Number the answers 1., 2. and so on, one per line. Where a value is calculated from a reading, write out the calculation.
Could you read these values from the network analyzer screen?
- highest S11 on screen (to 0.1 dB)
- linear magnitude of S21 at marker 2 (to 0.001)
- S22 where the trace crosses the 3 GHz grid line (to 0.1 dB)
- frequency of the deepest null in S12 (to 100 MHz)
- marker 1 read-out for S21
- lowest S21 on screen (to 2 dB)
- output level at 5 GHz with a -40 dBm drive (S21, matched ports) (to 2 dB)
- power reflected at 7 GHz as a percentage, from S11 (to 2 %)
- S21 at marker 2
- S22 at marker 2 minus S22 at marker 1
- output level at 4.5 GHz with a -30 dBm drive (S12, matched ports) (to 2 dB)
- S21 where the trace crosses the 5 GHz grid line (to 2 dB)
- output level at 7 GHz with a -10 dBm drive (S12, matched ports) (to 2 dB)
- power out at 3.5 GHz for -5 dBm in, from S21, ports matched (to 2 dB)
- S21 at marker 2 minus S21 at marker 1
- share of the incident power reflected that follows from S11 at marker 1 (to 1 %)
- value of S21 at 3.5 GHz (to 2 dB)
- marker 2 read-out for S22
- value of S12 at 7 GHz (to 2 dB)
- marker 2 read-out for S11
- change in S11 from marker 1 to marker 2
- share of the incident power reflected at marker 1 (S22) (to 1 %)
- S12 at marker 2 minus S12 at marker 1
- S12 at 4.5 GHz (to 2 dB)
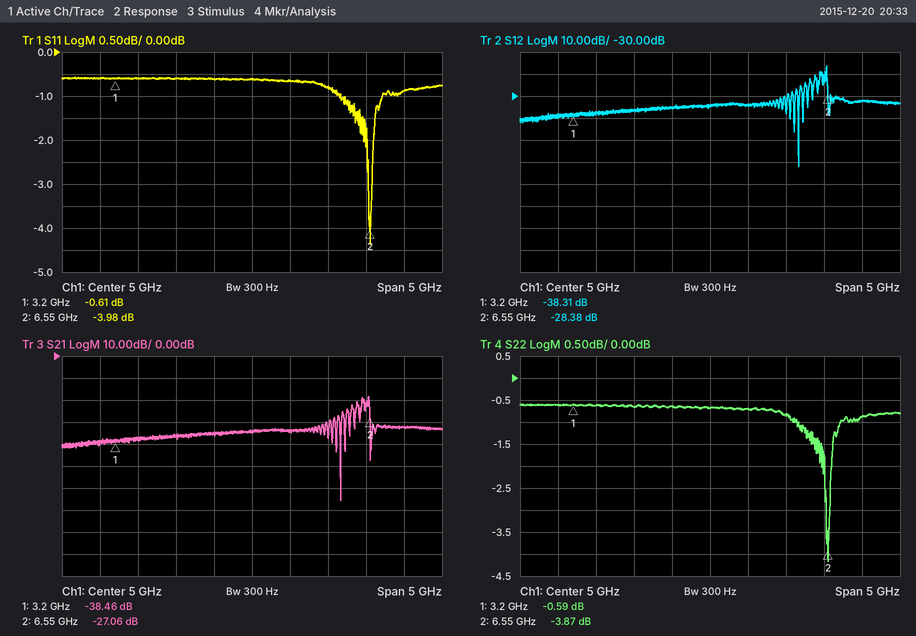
1. -0.6 dB
2. 10^(-27.06/20) ≈ 0.044
3. -0.6 dB
4. 6.2 GHz
5. -38.46 dB
6. -66 dB
7. -40 dBm + (-34 dB) = -74 dBm
8. 10^(-0.9/10) ≈ 81.3 %, so 82 % to the nearest 2 %
9. -27.06 dB
10. -3.87 − (-0.59) = -3.28 dB
11. -30 dBm + (-36 dB) = -66 dBm
12. -34 dB
13. -10 dBm + (-32 dB) = -42 dBm
14. -5 dBm + (-38 dB) = -42 dBm
15. -27.06 − (-38.46) = 11.40 dB
16. 10^(-0.61/10) ≈ 87 %
17. -38 dB
18. -3.87 dB
19. -32 dB
20. -3.98 dB
21. -3.98 − (-0.61) = -3.37 dB
22. 10^(-0.59/10) ≈ 87 %
23. -28.38 − (-38.31) = 9.93 dB
24. -36 dB
